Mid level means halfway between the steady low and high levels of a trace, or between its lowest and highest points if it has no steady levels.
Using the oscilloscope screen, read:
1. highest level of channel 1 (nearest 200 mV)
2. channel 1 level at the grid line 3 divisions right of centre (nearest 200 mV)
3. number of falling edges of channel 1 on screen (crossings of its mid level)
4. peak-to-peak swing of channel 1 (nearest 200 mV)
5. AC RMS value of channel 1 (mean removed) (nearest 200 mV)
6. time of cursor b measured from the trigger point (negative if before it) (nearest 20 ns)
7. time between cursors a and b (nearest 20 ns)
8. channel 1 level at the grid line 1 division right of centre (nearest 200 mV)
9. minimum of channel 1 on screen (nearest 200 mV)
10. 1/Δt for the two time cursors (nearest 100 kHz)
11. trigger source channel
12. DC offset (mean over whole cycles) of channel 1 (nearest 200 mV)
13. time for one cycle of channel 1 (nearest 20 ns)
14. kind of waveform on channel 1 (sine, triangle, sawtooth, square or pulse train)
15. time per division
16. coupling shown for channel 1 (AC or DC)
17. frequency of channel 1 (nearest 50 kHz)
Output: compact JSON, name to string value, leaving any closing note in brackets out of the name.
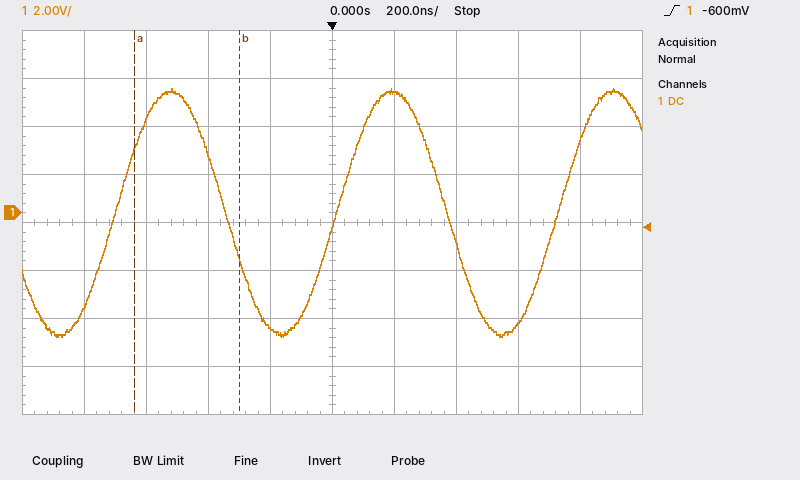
{"highest level of channel 1": "5.2 V", "channel 1 level at the grid line 3 divisions right of centre": "-4.6 V", "number of falling edges of channel 1 on screen": "2", "peak-to-peak swing of channel 1": "10.4 V", "AC RMS value of channel 1 (mean removed)": "3.6 V", "time of cursor b measured from the trigger point (negative if before it)": "-300 ns", "time between cursors a and b": "340 ns", "channel 1 level at the grid line 1 division right of centre": "5.0 V", "minimum of channel 1 on screen": "-5.2 V", "1/Δt for the two time cursors": "2.9 MHz", "trigger source channel": "channel 1", "DC offset (mean over whole cycles) of channel 1": "0.0 V", "time for one cycle of channel 1": "720 ns", "kind of waveform on channel 1": "sine", "time per division": "200 ns", "coupling shown for channel 1": "DC", "frequency of channel 1": "1.40 MHz"}
